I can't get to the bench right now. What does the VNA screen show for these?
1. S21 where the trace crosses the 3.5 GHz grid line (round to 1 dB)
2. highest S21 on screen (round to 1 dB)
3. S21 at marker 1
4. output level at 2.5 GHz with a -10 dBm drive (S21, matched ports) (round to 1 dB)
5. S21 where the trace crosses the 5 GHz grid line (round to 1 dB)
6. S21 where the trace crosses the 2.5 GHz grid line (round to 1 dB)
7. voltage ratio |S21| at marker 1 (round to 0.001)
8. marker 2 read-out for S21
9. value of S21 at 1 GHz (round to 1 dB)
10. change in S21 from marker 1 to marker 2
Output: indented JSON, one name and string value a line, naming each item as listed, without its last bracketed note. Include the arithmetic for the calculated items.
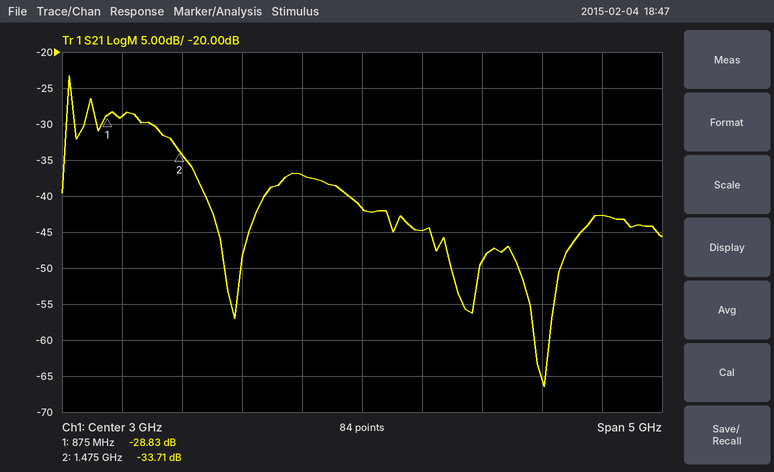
{
  "S21 where the trace crosses the 3.5 GHz grid line": "-45 dB",
  "highest S21 on screen": "-23 dB",
  "S21 at marker 1": "-28.83 dB",
  "output level at 2.5 GHz with a -10 dBm drive (S21, matched ports)": "-10 dBm + (-37 dB) = -47 dBm",
  "S21 where the trace crosses the 5 GHz grid line": "-43 dB",
  "S21 where the trace crosses the 2.5 GHz grid line": "-37 dB",
  "voltage ratio |S21| at marker 1": "10^(-28.83/20) ≈ 0.036",
  "marker 2 read-out for S21": "-33.71 dB",
  "value of S21 at 1 GHz": "-29 dB",
  "change in S21 from marker 1 to marker 2": "-33.71 − (-28.83) = -4.88 dB"
}
